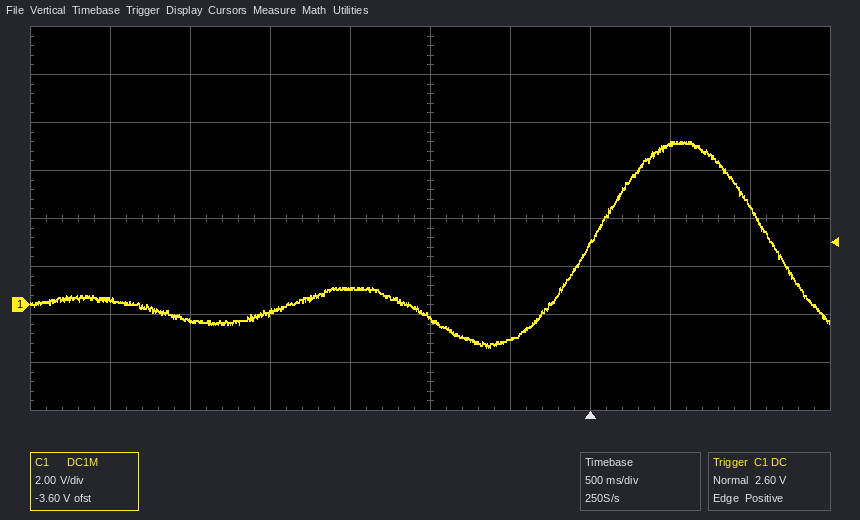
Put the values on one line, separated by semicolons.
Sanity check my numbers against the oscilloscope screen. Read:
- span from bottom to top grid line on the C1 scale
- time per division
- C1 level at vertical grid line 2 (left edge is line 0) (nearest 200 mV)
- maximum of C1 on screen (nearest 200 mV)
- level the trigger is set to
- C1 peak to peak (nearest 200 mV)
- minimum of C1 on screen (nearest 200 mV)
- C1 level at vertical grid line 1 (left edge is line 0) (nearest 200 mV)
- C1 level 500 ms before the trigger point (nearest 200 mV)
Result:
16 V; 500 ms; -600 mV; 6.8 V; 2.60 V; 8.6 V; -1.8 V; 200 mV; -1.4 V
